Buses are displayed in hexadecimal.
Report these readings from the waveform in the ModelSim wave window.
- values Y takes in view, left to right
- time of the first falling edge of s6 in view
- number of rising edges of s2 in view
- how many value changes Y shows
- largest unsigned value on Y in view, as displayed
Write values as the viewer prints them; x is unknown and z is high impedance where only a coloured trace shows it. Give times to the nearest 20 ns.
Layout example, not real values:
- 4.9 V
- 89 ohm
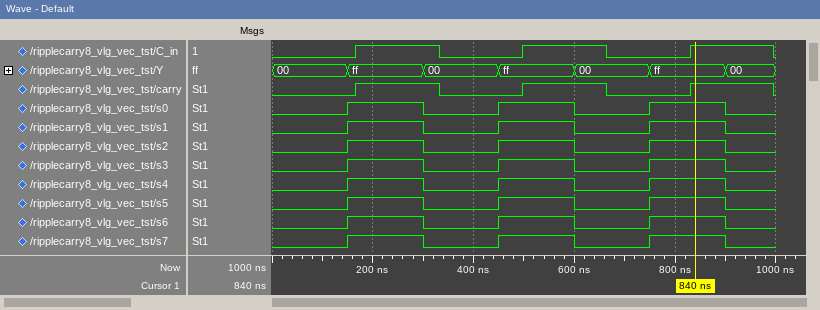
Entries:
- 00, ff, 00, ff, 00, ff, 00
- 300 ns
- 3
- 6
- ff
